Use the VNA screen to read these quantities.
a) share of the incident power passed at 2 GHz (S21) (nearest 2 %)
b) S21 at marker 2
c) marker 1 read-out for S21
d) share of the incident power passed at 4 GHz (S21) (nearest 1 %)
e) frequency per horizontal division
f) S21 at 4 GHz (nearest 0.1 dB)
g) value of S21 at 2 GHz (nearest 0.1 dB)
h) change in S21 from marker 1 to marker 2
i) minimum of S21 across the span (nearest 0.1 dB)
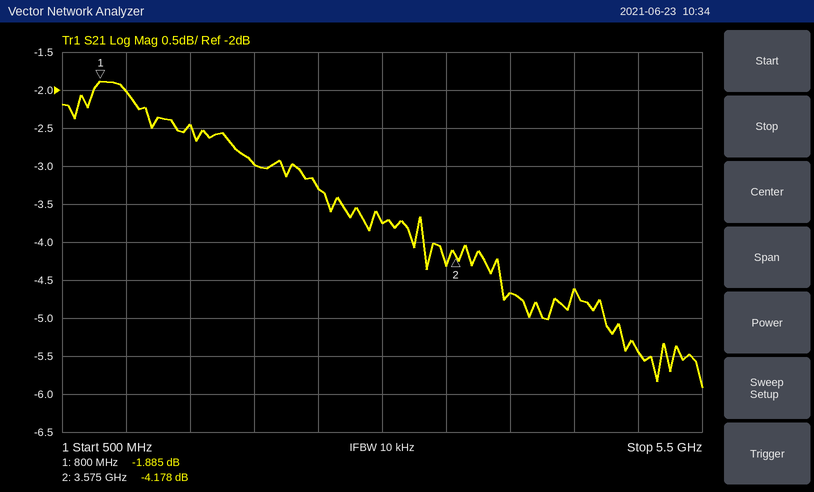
50 %
-4.178 dB
-1.885 dB
34 %
500 MHz
-4.7 dB
-3.0 dB
-2.293 dB
-5.9 dB
